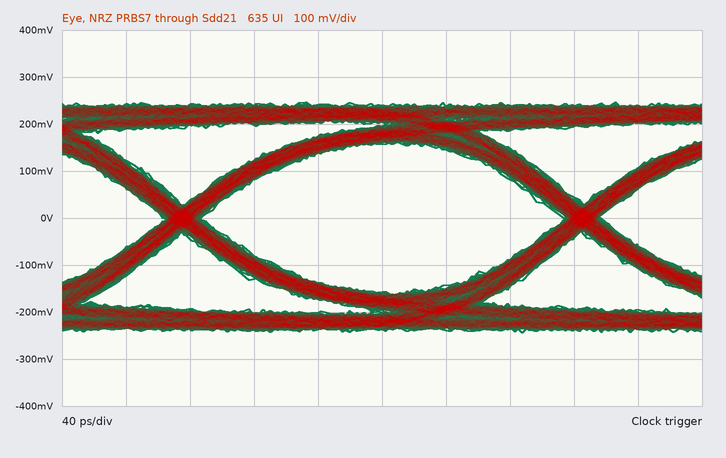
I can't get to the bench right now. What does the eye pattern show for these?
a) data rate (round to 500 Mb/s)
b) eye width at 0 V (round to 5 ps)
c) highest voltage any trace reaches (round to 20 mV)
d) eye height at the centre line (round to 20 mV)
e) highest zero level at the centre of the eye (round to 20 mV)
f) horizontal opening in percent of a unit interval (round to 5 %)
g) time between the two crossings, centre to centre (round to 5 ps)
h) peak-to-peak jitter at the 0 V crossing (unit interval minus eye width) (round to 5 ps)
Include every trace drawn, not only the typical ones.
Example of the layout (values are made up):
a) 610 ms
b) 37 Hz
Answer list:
a) 4.0 Gb/s
b) 225 ps
c) 240 mV
d) 320 mV
e) -160 mV
f) 90 %
g) 250 ps
h) 25 ps
